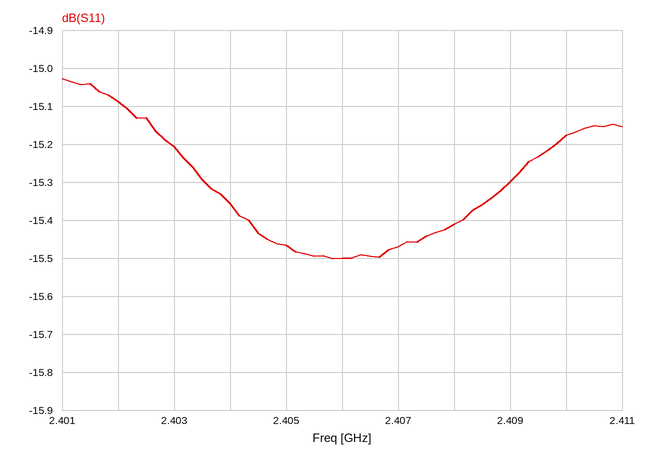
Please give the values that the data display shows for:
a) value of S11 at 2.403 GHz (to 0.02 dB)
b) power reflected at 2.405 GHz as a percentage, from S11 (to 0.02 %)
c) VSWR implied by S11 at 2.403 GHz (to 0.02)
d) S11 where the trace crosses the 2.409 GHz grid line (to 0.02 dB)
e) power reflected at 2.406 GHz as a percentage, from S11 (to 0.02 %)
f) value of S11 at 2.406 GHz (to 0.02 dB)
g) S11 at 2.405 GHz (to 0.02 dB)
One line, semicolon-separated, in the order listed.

-15.20 dB; 2.84 %; 1.42; -15.30 dB; 2.82 %; -15.50 dB; -15.46 dB
